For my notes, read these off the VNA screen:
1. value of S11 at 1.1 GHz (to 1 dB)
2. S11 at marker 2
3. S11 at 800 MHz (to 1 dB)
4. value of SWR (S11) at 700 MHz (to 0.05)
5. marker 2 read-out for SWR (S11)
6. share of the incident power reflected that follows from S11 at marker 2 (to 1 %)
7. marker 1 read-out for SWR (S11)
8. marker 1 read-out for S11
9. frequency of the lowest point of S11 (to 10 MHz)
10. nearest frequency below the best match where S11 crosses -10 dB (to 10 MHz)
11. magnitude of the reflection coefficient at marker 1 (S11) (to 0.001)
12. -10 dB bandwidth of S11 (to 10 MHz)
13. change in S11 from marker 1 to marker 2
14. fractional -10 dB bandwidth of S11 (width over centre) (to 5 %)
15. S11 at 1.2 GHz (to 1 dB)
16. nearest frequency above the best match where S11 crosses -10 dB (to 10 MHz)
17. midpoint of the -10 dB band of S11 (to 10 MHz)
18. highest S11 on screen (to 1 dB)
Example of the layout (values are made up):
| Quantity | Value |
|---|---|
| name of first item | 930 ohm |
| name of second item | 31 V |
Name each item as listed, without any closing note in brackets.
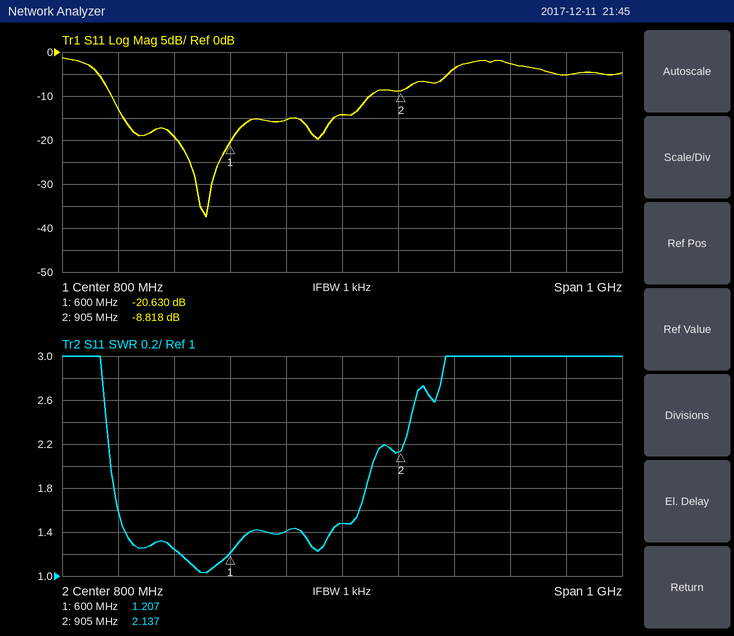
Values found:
| Quantity | Value |
|---|---|
| value of S11 at 1.1 GHz | -3 dB |
| S11 at marker 2 | -8.818 dB |
| S11 at 800 MHz | -14 dB |
| value of SWR (S11) at 700 MHz | 1.40 |
| marker 2 read-out for SWR | 2.137 |
| share of the incident power reflected that follows from S11 at marker 2 | 13 % |
| marker 1 read-out for SWR | 1.207 |
| marker 1 read-out for S11 | -20.630 dB |
| frequency of the lowest point of S11 | 560 MHz |
| nearest frequency below the best match where S11 crosses -10 dB | 390 MHz |
| magnitude of the reflection coefficient at marker 1 (S11) | 0.093 |
| -10 dB bandwidth of S11 | 460 MHz |
| change in S11 from marker 1 to marker 2 | 11.812 dB |
| fractional -10 dB bandwidth of S11 (width over centre) | 75 % |
| S11 at 1.2 GHz | -5 dB |
| nearest frequency above the best match where S11 crosses -10 dB | 850 MHz |
| midpoint of the -10 dB band of S11 | 620 MHz |
| highest S11 on screen | -1 dB |
